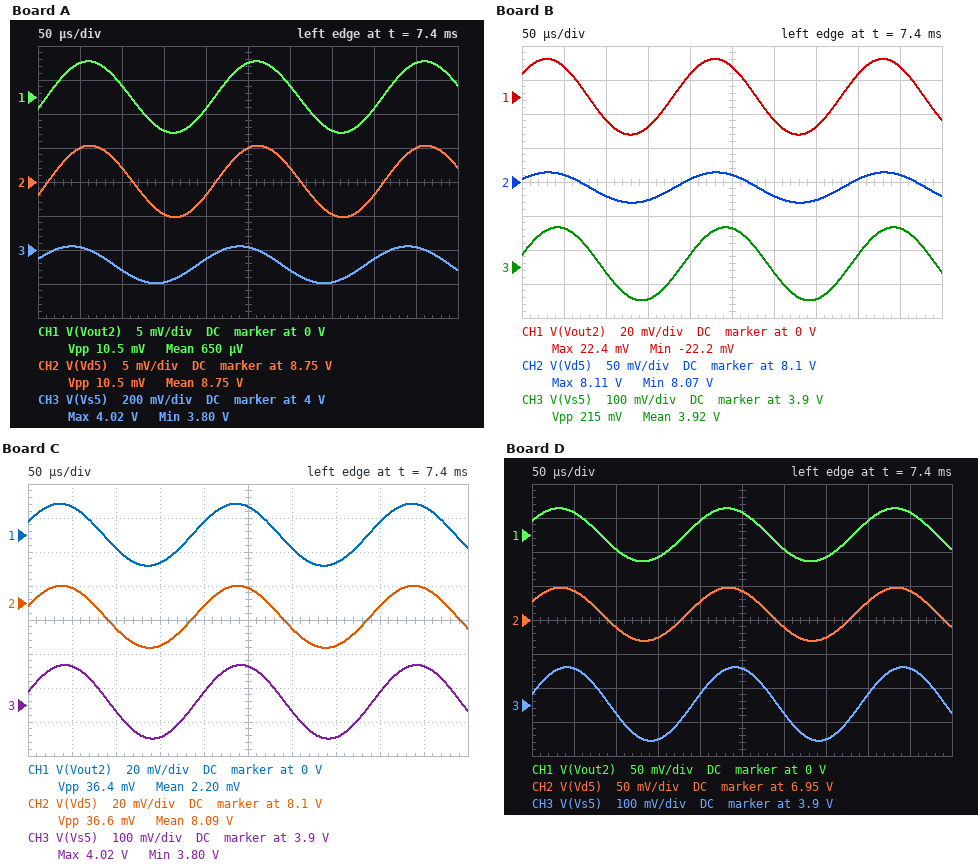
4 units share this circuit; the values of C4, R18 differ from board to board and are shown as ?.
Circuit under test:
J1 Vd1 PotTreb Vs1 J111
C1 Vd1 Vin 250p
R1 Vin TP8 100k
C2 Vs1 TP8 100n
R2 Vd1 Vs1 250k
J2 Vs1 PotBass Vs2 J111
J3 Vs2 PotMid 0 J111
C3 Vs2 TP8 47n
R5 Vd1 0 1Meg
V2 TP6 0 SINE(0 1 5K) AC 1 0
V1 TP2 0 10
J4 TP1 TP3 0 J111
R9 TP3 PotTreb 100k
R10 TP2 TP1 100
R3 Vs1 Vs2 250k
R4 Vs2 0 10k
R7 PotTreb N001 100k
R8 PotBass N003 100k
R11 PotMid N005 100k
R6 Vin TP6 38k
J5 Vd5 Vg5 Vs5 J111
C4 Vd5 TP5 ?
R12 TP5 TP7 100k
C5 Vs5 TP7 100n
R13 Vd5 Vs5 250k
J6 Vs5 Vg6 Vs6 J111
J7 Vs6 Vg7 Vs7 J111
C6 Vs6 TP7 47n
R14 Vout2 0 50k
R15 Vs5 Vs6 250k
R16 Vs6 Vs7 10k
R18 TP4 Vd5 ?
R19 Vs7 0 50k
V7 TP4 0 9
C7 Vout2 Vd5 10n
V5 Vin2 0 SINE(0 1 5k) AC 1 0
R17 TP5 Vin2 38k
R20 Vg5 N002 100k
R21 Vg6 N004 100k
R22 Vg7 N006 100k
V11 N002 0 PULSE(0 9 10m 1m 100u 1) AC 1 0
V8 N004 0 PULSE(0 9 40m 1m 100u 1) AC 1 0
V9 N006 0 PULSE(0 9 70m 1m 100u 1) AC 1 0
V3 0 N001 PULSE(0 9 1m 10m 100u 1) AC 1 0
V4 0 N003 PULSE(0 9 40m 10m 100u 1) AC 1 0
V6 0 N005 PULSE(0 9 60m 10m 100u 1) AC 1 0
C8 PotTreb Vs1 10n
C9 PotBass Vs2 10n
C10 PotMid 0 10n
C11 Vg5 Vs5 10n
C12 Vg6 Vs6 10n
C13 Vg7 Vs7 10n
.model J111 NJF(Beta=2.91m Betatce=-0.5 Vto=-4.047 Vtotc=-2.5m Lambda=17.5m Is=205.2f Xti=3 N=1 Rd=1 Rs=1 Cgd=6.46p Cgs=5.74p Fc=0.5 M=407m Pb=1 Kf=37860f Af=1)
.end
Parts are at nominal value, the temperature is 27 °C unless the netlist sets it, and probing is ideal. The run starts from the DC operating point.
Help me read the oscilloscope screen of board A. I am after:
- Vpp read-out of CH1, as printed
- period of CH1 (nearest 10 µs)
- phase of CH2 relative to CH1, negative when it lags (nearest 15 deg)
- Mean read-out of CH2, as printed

10.5 mV
200 µs
0 deg
8.75 V
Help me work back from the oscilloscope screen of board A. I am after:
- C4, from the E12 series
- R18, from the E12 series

82 pF
3.3 kΩ
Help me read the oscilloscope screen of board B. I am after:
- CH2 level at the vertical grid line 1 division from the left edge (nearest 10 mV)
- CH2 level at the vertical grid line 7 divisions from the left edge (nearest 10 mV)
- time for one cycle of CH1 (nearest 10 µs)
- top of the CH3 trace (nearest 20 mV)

8.11 V
8.07 V
200 µs
4.02 V
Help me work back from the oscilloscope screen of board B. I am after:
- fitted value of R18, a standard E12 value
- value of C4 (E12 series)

12 kΩ
180 pF
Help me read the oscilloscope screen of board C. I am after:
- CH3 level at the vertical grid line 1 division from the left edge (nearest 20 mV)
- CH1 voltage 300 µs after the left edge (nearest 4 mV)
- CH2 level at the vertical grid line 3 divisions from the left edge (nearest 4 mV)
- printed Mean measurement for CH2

4.02 V
-8 mV
8.076 V
8.09 V
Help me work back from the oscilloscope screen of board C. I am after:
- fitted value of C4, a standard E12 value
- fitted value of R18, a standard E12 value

150 pF
12 kΩ
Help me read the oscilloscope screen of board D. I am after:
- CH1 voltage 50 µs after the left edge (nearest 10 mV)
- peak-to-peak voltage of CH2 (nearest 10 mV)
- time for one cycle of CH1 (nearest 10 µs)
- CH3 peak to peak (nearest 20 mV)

30 mV
80 mV
200 µs
220 mV
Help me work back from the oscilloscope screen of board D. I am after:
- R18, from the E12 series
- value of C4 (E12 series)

27 kΩ
180 pF
